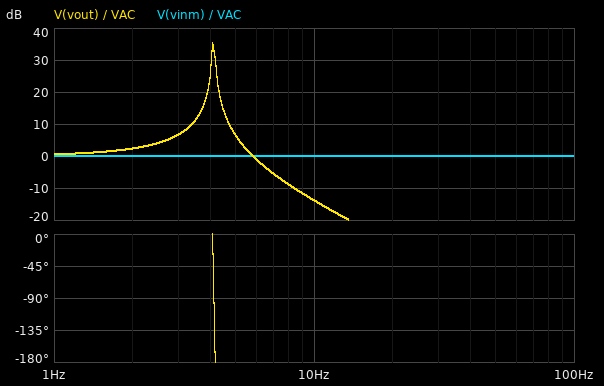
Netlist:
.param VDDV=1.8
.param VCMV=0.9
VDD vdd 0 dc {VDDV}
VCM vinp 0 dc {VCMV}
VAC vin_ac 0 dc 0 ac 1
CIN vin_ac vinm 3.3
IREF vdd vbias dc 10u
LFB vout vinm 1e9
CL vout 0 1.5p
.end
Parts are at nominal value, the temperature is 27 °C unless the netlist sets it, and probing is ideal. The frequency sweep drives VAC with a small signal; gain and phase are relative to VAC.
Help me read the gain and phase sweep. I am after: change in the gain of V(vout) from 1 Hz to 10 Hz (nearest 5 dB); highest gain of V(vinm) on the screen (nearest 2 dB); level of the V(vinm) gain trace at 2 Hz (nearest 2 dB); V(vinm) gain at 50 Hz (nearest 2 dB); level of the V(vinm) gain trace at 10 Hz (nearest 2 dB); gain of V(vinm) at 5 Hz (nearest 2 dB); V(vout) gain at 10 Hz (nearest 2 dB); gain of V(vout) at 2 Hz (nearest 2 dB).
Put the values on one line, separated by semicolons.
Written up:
-15 dB; 0 dB; 0 dB; 0 dB; 0 dB; 0 dB; -14 dB; 2 dB
